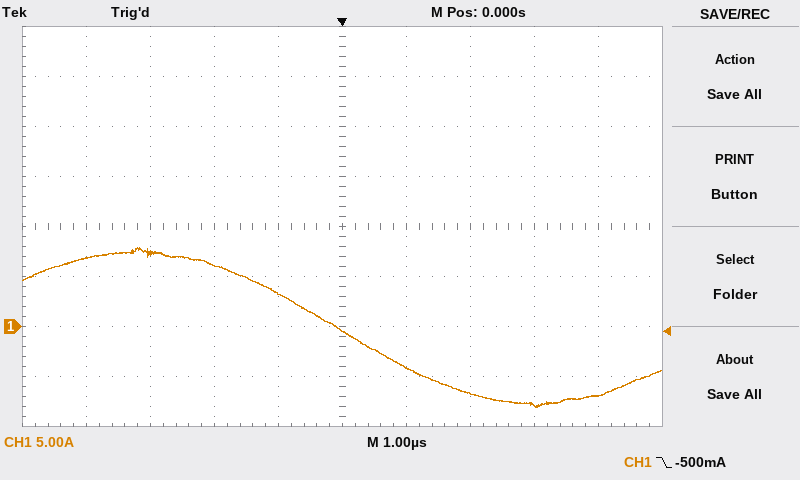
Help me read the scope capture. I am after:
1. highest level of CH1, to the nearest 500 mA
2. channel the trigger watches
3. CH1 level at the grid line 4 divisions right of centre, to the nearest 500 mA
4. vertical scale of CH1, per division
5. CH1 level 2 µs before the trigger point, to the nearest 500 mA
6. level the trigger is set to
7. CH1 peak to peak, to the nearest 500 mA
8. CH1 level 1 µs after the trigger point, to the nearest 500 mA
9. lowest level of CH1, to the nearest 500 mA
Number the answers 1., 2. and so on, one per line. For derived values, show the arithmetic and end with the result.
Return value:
1. 8.0 A
2. CH1
3. -7.0 A
4. 5 A
5. 6.0 A
6. -500 mA
7. 8.0 A − (-8.0 A) = 16.0 A
8. -4.0 A
9. -8.0 A
